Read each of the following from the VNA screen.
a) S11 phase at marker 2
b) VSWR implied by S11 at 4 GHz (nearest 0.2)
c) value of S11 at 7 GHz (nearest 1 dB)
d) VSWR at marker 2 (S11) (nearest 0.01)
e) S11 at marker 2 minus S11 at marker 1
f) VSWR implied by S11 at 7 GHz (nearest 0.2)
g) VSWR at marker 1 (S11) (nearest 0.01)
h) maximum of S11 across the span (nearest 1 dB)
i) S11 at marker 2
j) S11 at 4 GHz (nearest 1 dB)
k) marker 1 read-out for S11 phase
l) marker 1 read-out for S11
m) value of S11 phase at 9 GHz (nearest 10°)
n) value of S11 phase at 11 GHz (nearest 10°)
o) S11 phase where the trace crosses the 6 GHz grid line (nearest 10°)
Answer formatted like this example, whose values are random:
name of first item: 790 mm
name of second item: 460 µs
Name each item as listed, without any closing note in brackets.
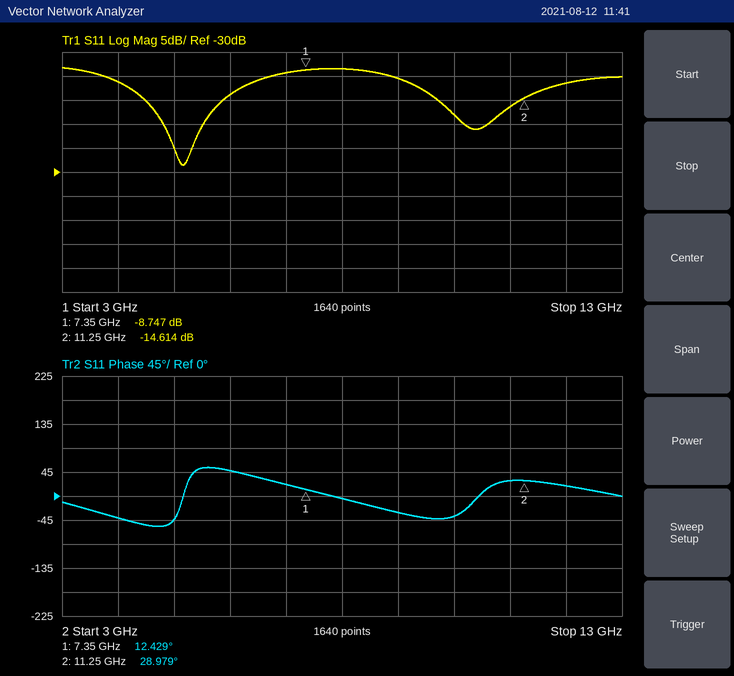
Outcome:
S11 phase at marker 2: 28.979°
VSWR implied by S11 at 4 GHz: 1.8
value of S11 at 7 GHz: -9 dB
VSWR at marker 2 (S11): 1.46
S11 at marker 2 minus S11 at marker 1: -5.867 dB
VSWR implied by S11 at 7 GHz: 2.0
VSWR at marker 1 (S11): 2.15
maximum of S11 across the span: -8 dB
S11 at marker 2: -14.614 dB
S11 at 4 GHz: -11 dB
marker 1 read-out for S11 phase: 12.429°
marker 1 read-out for S11: -8.747 dB
value of S11 phase at 9 GHz: -30°
value of S11 phase at 11 GHz: 30°
S11 phase where the trace crosses the 6 GHz grid line: 50°
